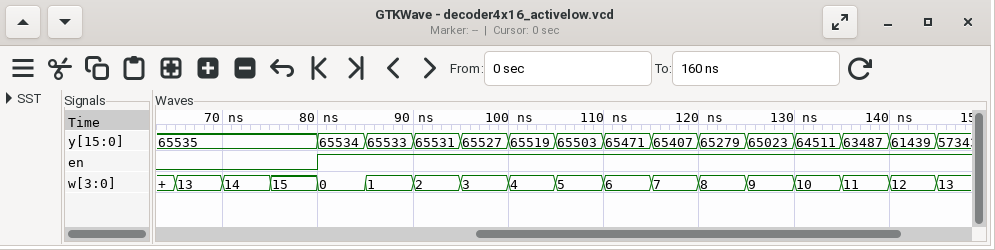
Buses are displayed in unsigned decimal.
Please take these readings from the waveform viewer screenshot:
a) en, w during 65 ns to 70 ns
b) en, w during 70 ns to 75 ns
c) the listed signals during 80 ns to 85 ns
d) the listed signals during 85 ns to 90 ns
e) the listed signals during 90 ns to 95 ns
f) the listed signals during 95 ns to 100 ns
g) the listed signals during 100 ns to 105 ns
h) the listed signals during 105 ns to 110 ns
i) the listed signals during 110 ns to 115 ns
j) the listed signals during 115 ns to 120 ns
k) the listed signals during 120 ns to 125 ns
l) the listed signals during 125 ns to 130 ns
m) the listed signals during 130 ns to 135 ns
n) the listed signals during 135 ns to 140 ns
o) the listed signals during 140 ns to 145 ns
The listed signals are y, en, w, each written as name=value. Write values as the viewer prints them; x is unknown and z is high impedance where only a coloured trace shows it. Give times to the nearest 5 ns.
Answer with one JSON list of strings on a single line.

["en=0, w=13", "en=0, w=14", "y=65534, en=1, w=0", "y=65533, en=1, w=1", "y=65531, en=1, w=2", "y=65527, en=1, w=3", "y=65519, en=1, w=4", "y=65503, en=1, w=5", "y=65471, en=1, w=6", "y=65407, en=1, w=7", "y=65279, en=1, w=8", "y=65023, en=1, w=9", "y=64511, en=1, w=10", "y=63487, en=1, w=11", "y=61439, en=1, w=12"]
